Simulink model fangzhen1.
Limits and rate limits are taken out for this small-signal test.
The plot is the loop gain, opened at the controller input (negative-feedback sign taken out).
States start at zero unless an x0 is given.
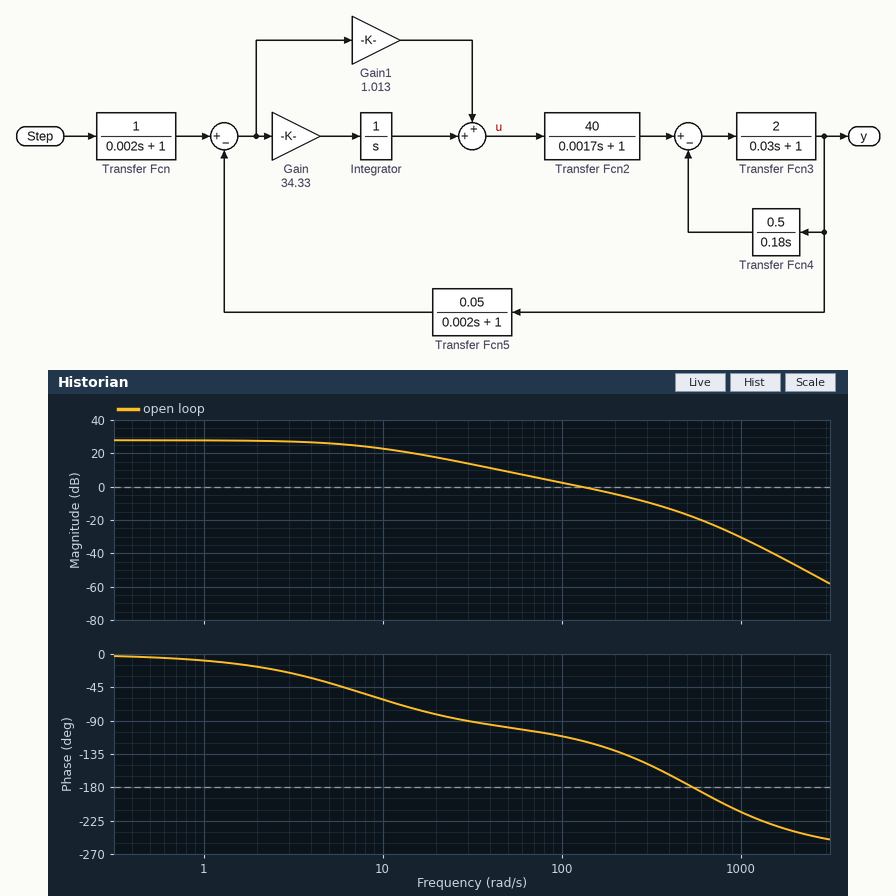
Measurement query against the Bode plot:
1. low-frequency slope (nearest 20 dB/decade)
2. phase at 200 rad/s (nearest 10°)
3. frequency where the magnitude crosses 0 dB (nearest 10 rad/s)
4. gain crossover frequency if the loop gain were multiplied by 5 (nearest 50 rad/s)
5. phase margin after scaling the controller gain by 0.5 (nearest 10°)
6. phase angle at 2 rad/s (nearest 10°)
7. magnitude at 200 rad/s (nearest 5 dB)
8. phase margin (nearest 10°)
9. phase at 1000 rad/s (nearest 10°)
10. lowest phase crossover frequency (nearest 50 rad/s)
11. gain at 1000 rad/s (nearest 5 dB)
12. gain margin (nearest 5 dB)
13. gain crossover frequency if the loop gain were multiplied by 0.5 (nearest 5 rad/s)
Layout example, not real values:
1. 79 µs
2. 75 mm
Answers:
1. 0 dB/decade
2. -130°
3. 130 rad/s
4. 400 rad/s
5. 80°
6. -20°
7. -5 dB
8. 60°
9. -210°
10. 550 rad/s
11. -30 dB
12. 20 dB
13. 70 rad/s
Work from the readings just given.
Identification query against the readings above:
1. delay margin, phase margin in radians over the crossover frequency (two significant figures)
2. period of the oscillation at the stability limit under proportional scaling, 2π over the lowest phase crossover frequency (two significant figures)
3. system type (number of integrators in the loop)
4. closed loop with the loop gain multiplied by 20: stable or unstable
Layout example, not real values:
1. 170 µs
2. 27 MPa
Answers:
1. 0.0081 s
2. 0.011 s
3. 0
4. unstable
